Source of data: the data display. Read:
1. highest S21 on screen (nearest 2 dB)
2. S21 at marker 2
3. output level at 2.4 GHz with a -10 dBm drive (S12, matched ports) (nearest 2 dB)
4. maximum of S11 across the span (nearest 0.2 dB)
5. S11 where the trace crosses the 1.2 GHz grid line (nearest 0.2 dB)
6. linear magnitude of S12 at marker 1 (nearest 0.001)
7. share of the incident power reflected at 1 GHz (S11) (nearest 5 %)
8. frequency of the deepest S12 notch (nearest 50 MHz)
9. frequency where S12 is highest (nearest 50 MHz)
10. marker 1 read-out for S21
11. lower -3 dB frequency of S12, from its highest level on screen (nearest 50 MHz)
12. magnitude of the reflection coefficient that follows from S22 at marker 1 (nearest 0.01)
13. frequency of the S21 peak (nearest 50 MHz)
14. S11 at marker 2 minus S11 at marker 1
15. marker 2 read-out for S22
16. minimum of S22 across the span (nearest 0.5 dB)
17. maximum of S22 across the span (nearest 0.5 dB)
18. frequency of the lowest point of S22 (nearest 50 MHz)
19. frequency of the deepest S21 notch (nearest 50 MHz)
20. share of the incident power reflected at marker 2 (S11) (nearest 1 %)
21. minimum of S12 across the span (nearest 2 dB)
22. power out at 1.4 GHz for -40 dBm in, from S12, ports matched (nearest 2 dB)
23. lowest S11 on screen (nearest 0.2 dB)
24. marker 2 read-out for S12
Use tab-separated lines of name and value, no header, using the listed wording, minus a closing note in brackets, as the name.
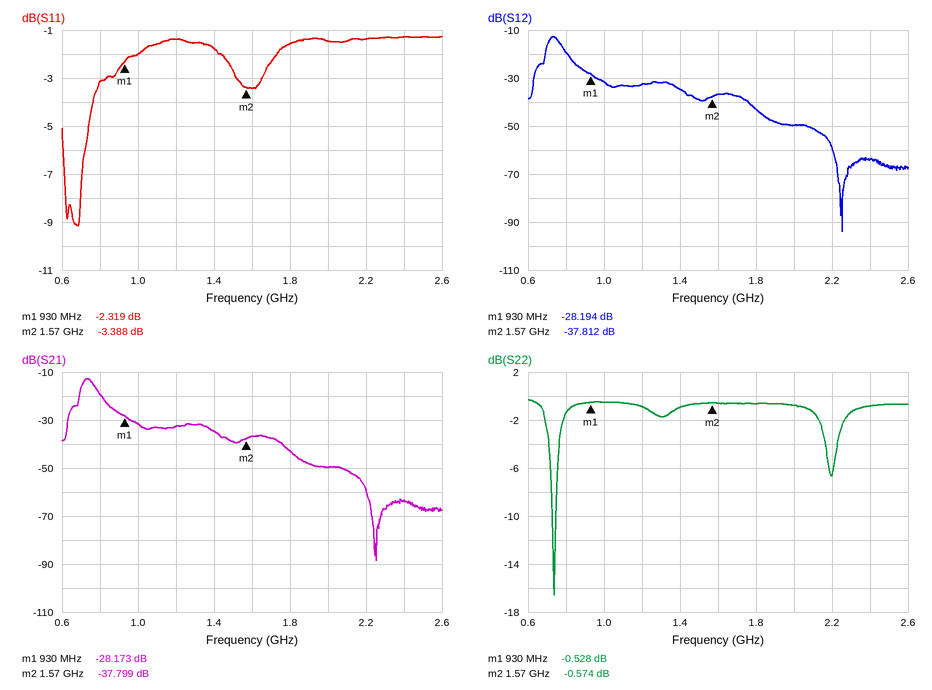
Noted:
highest S21 on screen	-12 dB
S21 at marker 2	-37.799 dB
output level at 2.4 GHz with a -10 dBm drive (S12, matched ports)	-74 dBm
maximum of S11 across the span	-1.2 dB
S11 where the trace crosses the 1.2 GHz grid line	-1.4 dB
linear magnitude of S12 at marker 1	0.039
share of the incident power reflected at 1 GHz (S11)	65 %
frequency of the deepest S12 notch	2.25 GHz
frequency where S12 is highest	750 MHz
marker 1 read-out for S21	-28.173 dB
lower -3 dB frequency of S12, from its highest level on screen	700 MHz
magnitude of the reflection coefficient that follows from S22 at marker 1	0.94
frequency of the S21 peak	750 MHz
S11 at marker 2 minus S11 at marker 1	-1.069 dB
marker 2 read-out for S22	-0.574 dB
minimum of S22 across the span	-16.5 dB
maximum of S22 across the span	-0.5 dB
frequency of the lowest point of S22	750 MHz
frequency of the deepest S21 notch	2.25 GHz
share of the incident power reflected at marker 2 (S11)	46 %
minimum of S12 across the span	-94 dB
power out at 1.4 GHz for -40 dBm in, from S12, ports matched	-74 dBm
lowest S11 on screen	-9.2 dB
marker 2 read-out for S12	-37.812 dB
